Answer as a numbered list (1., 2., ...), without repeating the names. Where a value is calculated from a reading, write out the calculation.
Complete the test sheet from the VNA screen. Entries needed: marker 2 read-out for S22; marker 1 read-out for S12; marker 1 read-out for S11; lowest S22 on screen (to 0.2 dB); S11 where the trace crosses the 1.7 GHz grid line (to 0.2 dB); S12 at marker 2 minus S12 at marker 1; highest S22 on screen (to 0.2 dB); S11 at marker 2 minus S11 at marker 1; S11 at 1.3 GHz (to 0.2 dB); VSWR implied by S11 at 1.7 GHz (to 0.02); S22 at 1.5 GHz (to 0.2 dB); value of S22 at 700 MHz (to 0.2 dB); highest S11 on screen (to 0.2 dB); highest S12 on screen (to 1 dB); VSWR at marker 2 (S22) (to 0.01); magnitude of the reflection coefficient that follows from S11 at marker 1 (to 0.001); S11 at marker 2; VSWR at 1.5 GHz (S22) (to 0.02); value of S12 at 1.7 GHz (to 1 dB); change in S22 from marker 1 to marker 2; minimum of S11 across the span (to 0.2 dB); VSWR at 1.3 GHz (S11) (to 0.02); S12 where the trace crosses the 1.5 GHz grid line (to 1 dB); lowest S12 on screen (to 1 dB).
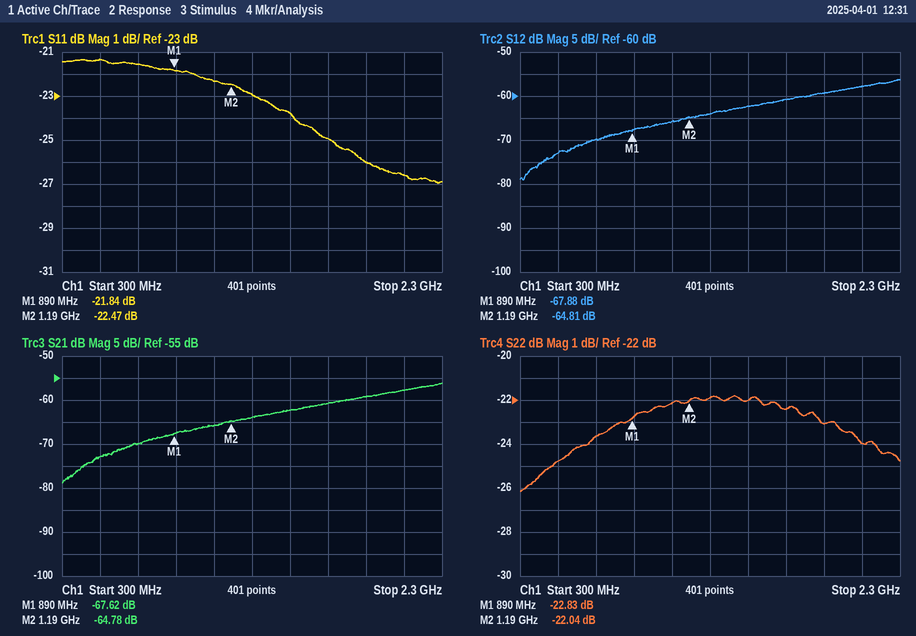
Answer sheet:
1. -22.04 dB
2. -67.88 dB
3. -21.84 dB
4. -26.2 dB
5. -25.0 dB
6. -64.81 − (-67.88) = 3.07 dB
7. -21.8 dB
8. -22.47 − (-21.84) = -0.63 dB
9. -23.0 dB
10. |Γ| = 10^(-25/20) = 0.0562; VSWR = (1 + 0.0562)/(1 − 0.0562) ≈ 1.12
11. -22.0 dB
12. -23.6 dB
13. -21.4 dB
14. -56 dB
15. (1 + 0.0791)/(1 − 0.0791) ≈ 1.17
16. 10^(-21.84/20) ≈ 0.081
17. -22.47 dB
18. |Γ| = 10^(-22/20) = 0.0794; VSWR = (1 + 0.0794)/(1 − 0.0794) ≈ 1.17, so 1.18 to the nearest 0.02
19. -61 dB
20. -22.04 − (-22.83) = 0.79 dB
21. -27.0 dB
22. |Γ| = 10^(-23/20) = 0.0708; VSWR = (1 + 0.0708)/(1 − 0.0708) ≈ 1.15, so 1.16 to the nearest 0.02
23. -62 dB
24. -79 dB
